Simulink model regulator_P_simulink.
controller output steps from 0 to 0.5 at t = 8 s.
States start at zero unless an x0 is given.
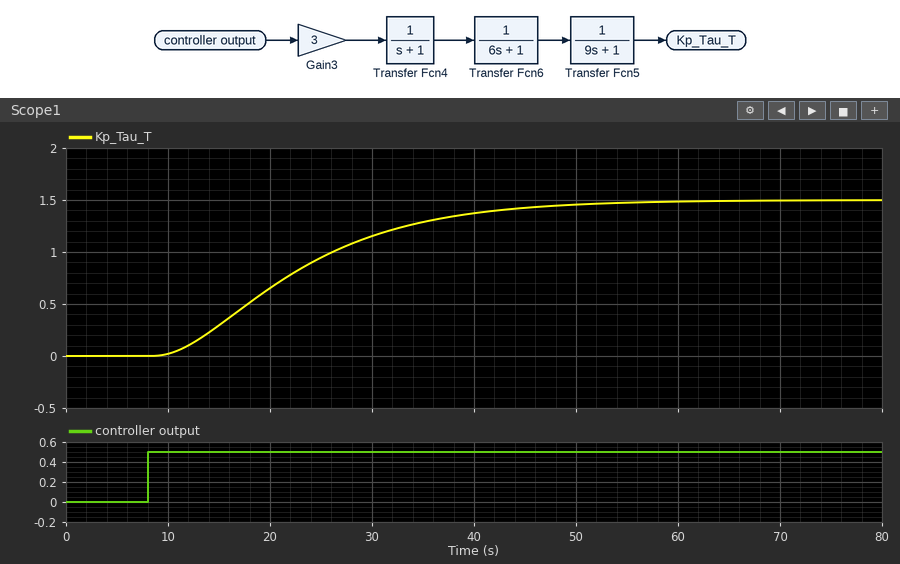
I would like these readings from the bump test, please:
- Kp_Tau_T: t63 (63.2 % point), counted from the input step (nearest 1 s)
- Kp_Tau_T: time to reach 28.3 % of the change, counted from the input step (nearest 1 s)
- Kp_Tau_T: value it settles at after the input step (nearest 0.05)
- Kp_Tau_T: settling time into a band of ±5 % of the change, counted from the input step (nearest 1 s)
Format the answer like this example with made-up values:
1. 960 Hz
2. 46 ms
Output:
1. 17 s
2. 9 s
3. 1.50
4. 37 s
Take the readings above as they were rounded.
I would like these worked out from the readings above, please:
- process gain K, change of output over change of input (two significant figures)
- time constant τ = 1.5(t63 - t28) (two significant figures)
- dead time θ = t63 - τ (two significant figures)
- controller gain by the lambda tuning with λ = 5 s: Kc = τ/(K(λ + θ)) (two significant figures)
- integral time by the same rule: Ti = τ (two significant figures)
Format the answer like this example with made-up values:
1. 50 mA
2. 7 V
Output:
1. 3.0
2. 12 s
3. 5.0 s
4. 0.40
5. 12 s
